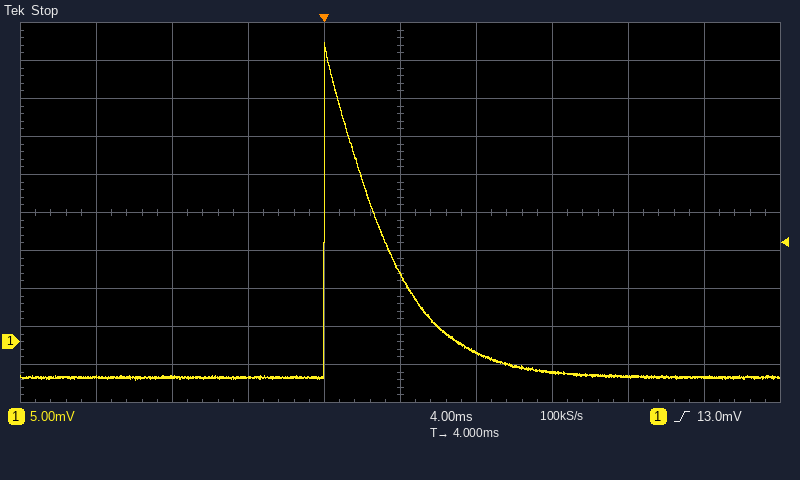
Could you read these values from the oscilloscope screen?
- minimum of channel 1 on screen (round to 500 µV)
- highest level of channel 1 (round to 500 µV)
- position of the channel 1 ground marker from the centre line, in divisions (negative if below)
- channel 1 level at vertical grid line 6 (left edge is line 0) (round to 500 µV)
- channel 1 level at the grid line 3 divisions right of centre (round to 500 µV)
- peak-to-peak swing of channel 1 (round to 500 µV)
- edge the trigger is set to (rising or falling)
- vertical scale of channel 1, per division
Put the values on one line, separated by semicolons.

-5.0 mV; 39.5 mV; -3.4 div; -1.5 mV; -4.5 mV; 44.5 mV; rising; 5 mV
